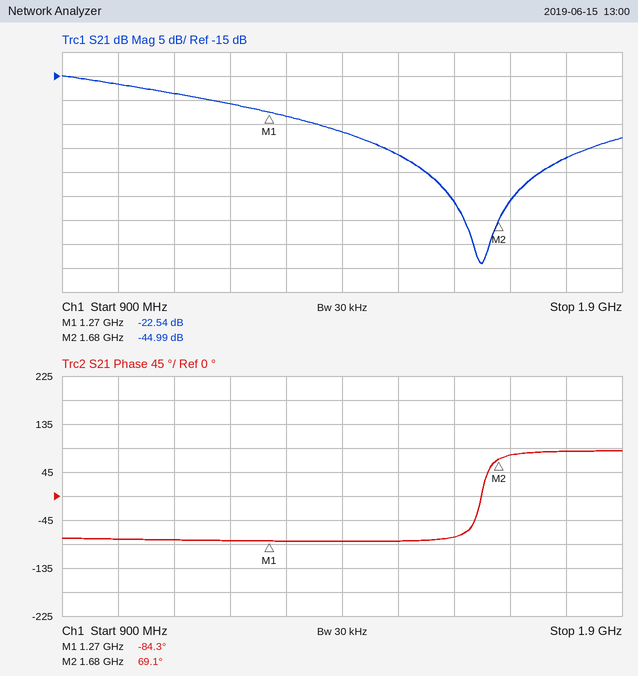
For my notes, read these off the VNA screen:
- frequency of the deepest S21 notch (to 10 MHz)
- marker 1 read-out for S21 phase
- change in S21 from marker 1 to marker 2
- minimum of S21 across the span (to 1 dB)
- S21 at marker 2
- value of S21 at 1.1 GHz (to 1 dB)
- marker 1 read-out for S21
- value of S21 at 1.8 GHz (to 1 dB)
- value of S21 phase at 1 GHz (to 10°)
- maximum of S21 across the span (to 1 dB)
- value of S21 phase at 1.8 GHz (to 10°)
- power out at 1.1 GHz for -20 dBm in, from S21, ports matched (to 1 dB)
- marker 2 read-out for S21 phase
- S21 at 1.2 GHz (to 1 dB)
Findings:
1.65 GHz
-84.3°
-22.45 dB
-54 dB
-44.99 dB
-19 dB
-22.54 dB
-32 dB
-80°
-15 dB
80°
-39 dBm
69.1°
-21 dB
